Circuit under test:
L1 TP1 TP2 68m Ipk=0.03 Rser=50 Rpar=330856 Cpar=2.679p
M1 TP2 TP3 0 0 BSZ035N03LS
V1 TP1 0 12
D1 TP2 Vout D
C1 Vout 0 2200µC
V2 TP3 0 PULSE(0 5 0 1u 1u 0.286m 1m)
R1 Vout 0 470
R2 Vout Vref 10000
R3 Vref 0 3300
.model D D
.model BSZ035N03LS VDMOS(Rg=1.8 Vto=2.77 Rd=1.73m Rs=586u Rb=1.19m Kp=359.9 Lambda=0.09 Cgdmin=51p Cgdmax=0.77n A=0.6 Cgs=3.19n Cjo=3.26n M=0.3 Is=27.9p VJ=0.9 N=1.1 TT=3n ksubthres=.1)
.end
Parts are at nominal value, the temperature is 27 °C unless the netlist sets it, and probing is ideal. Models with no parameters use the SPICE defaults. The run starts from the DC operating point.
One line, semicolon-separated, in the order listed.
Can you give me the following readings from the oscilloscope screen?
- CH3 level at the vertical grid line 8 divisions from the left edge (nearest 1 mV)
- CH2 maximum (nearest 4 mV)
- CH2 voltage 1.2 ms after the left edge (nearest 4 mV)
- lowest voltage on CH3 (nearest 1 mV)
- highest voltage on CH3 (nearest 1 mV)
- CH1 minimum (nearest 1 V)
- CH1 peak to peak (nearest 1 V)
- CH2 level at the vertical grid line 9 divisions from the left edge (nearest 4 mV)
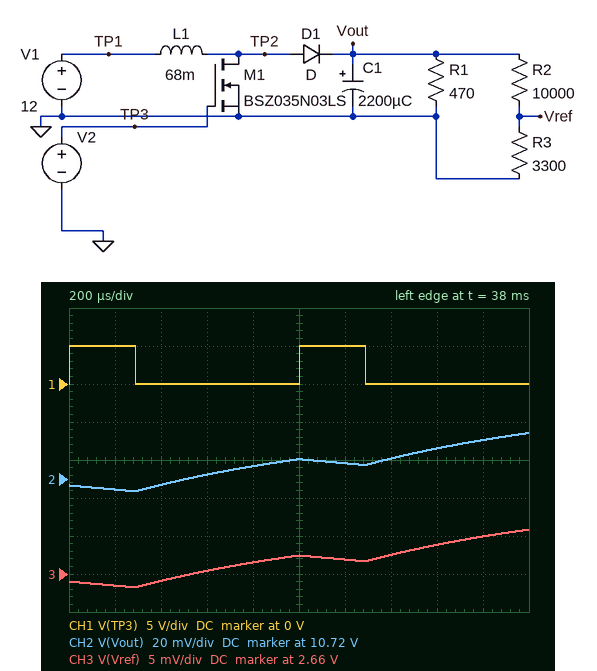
2.664 V; 10.744 V; 10.728 V; 2.658 V; 2.666 V; 0 V; 5 V; 10.740 V
